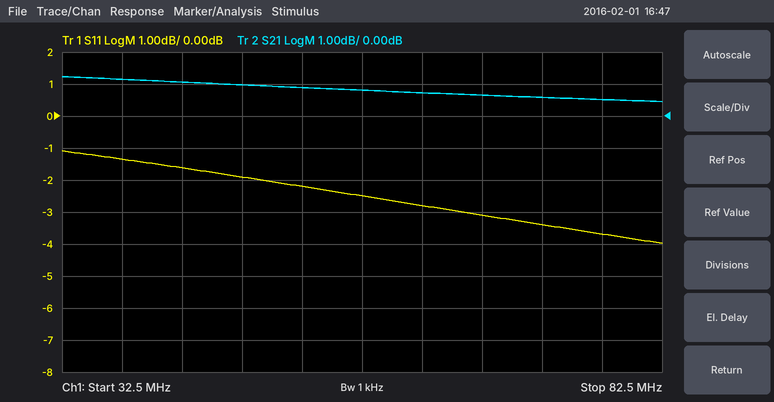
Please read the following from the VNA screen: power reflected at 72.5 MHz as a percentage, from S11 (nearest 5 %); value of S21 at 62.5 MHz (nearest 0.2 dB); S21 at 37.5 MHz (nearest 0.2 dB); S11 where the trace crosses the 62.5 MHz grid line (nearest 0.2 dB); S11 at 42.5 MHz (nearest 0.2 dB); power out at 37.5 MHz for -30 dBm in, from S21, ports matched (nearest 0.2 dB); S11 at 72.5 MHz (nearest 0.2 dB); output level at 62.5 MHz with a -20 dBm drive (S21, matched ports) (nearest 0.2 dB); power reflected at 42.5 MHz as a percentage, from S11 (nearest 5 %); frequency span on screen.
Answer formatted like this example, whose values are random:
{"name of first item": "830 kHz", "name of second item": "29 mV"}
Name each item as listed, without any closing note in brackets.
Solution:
{"power reflected at 72.5 MHz as a percentage, from S11": "45 %", "value of S21 at 62.5 MHz": "0.8 dB", "S21 at 37.5 MHz": "1.2 dB", "S11 where the trace crosses the 62.5 MHz grid line": "-2.8 dB", "S11 at 42.5 MHz": "-1.6 dB", "power out at 37.5 MHz for -30 dBm in, from S21, ports matched": "-28.8 dBm", "S11 at 72.5 MHz": "-3.4 dB", "output level at 62.5 MHz with a -20 dBm drive (S21, matched ports)": "-19.2 dBm", "power reflected at 42.5 MHz as a percentage, from S11": "70 %", "frequency span on screen": "50 MHz"}
